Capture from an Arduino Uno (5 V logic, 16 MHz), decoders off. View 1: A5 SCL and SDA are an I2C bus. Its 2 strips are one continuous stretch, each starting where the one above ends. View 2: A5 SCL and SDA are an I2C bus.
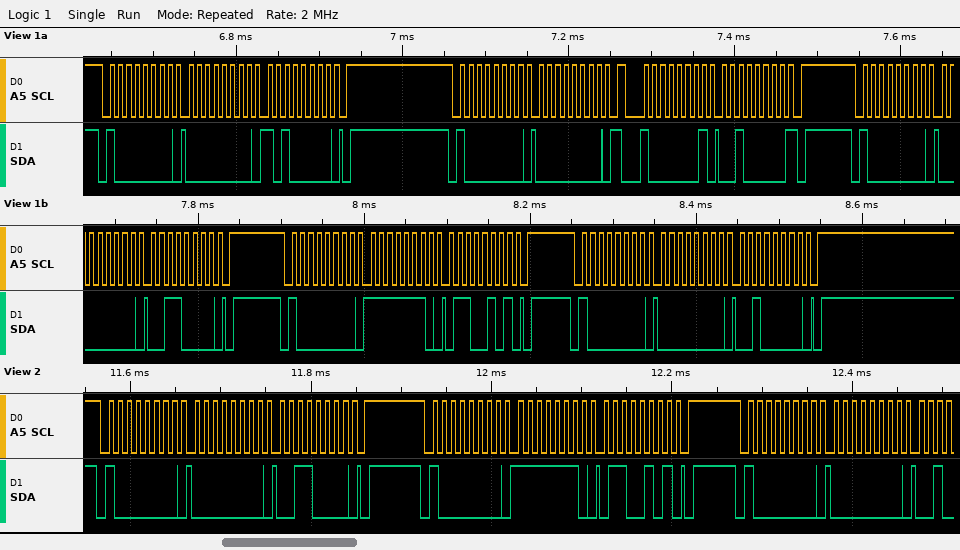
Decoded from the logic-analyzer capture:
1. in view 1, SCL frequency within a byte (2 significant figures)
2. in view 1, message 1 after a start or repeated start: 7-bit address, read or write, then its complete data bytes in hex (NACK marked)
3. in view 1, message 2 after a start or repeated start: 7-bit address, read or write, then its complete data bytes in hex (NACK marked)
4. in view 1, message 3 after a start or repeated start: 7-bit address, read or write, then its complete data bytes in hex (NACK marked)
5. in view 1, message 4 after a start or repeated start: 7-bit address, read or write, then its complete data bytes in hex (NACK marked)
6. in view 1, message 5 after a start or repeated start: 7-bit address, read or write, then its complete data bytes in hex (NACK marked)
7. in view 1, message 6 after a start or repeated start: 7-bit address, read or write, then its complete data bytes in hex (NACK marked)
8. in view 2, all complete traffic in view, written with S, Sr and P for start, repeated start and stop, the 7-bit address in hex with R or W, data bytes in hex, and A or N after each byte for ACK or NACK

100 kHz
0x40 write: 00 A0
0x40 write: 00
0x40 read: 20 NACK
0x40 write: 00 30
0x40 write: FE 65
0x40 write: 00 20
S 40W A 00 A 30 A P S 40W A FE A 65 A P S 40W A 00 A
